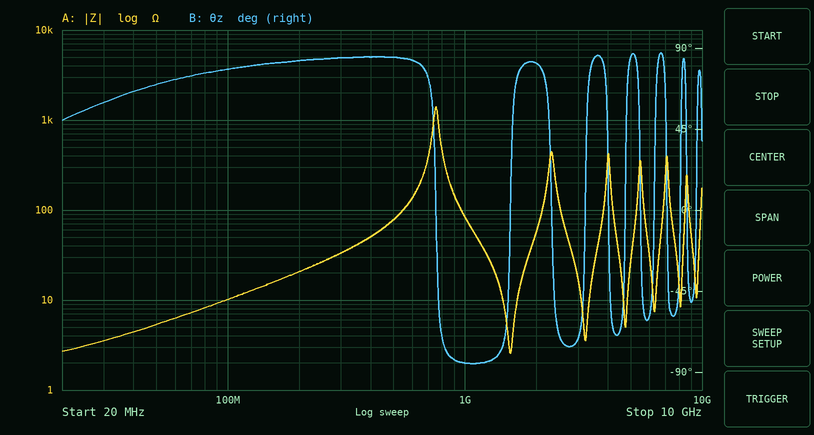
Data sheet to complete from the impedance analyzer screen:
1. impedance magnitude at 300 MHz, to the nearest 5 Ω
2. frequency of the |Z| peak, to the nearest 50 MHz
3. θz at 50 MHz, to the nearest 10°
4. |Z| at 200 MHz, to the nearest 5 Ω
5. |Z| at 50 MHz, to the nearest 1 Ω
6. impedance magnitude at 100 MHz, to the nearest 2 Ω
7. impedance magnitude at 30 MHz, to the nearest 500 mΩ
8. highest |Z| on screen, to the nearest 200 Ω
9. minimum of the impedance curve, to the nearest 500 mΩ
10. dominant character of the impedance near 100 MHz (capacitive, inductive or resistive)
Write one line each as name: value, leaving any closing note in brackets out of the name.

impedance magnitude at 300 MHz, to the nearest 5 Ω: 35 Ω
frequency of the |Z| peak, to the nearest 50 MHz: 750 MHz
θz at 50 MHz, to the nearest 10°: 70°
|Z| at 200 MHz, to the nearest 5 Ω: 20 Ω
|Z| at 50 MHz, to the nearest 1 Ω: 5 Ω
impedance magnitude at 100 MHz, to the nearest 2 Ω: 10 Ω
impedance magnitude at 30 MHz, to the nearest 500 mΩ: 3.5 Ω
highest |Z| on screen, to the nearest 200 Ω: 1.4 kΩ
minimum of the impedance curve, to the nearest 500 mΩ: 2.5 Ω
dominant character of the impedance near 100 MHz: inductive
